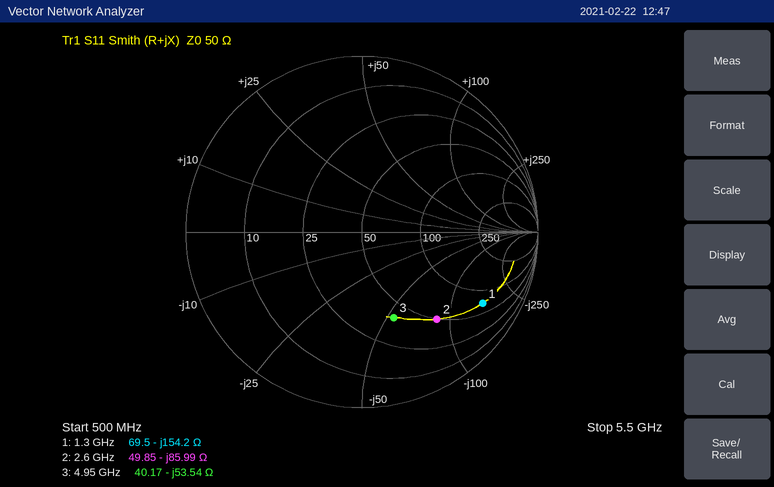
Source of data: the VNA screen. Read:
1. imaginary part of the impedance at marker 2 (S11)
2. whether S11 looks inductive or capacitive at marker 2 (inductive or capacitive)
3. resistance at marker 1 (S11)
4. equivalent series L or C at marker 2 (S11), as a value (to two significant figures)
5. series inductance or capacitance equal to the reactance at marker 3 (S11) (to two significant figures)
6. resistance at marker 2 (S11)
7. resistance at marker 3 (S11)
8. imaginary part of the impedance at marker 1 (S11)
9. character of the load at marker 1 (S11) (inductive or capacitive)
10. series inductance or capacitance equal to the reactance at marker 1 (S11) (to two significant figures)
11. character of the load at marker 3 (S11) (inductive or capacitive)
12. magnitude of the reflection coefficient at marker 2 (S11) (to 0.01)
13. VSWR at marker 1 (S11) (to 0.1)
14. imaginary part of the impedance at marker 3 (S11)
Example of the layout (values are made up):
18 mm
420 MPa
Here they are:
-85.99 Ω
capacitive
69.5 Ω
710 fF
600 fF
49.85 Ω
40.17 Ω
-154.2 Ω
capacitive
790 fF
capacitive
0.65
8.8
-53.54 Ω
